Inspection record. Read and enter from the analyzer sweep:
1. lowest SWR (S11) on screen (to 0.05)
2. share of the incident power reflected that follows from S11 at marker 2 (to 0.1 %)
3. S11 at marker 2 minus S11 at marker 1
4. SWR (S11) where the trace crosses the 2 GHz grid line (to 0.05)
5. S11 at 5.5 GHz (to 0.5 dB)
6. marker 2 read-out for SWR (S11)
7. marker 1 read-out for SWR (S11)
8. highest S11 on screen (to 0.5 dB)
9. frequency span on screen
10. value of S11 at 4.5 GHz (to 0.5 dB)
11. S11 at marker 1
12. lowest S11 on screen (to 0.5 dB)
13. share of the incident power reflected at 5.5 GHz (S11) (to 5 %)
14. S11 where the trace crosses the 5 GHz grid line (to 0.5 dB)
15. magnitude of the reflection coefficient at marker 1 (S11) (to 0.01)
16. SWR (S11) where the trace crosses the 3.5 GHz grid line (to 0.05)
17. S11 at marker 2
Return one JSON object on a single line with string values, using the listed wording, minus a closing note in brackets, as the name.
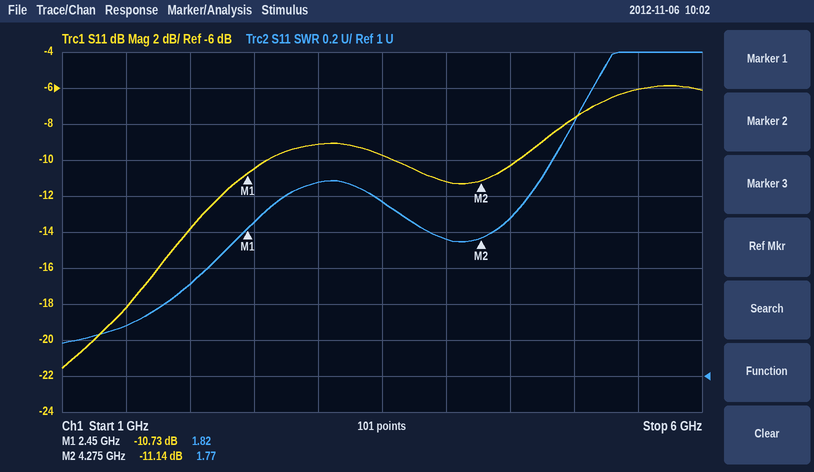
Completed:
{"lowest SWR (S11) on screen": "1.20", "share of the incident power reflected that follows from S11 at marker 2": "7.7 %", "S11 at marker 2 minus S11 at marker 1": "-0.41 dB", "SWR (S11) where the trace crosses the 2 GHz grid line": "1.50", "S11 at 5.5 GHz": "-6.0 dB", "marker 2 read-out for SWR": "1.77", "marker 1 read-out for SWR": "1.82", "highest S11 on screen": "-6.0 dB", "frequency span on screen": "5 GHz", "value of S11 at 4.5 GHz": "-10.5 dB", "S11 at marker 1": "-10.73 dB", "lowest S11 on screen": "-21.5 dB", "share of the incident power reflected at 5.5 GHz (S11)": "25 %", "S11 where the trace crosses the 5 GHz grid line": "-7.5 dB", "magnitude of the reflection coefficient at marker 1 (S11)": "0.29", "SWR (S11) where the trace crosses the 3.5 GHz grid line": "1.95", "S11 at marker 2": "-11.14 dB"}
